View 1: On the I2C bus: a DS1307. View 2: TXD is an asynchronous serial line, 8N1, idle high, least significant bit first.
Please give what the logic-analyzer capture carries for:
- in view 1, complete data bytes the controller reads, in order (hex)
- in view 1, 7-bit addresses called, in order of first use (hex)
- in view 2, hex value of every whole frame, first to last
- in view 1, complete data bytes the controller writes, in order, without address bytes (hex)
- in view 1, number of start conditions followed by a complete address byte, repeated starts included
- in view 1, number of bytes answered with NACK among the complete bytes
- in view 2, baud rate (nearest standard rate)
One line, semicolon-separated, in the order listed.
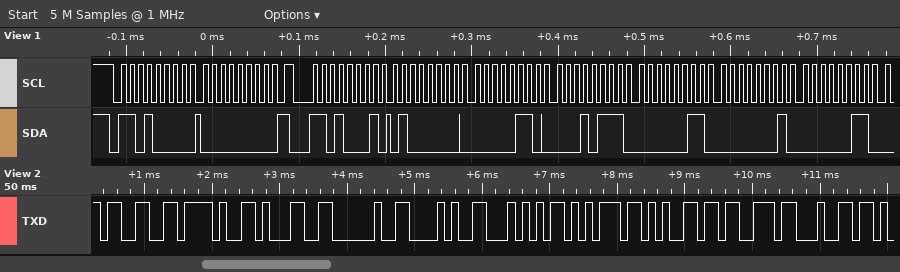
40 06 17 03 01 03; 0x68; 33 2F 31 20 28 54 75 65 73 64; 00; 2; 0; 9600 baud
